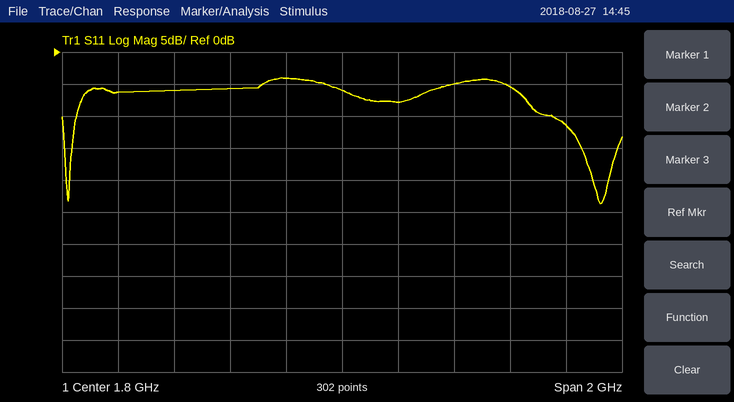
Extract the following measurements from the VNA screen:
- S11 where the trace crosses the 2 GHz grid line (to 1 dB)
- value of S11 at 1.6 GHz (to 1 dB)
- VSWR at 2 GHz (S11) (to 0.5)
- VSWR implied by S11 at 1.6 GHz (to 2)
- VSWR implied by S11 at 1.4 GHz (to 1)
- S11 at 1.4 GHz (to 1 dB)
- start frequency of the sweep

-8 dB
-4 dB
2.5
4
3
-6 dB
800 MHz
